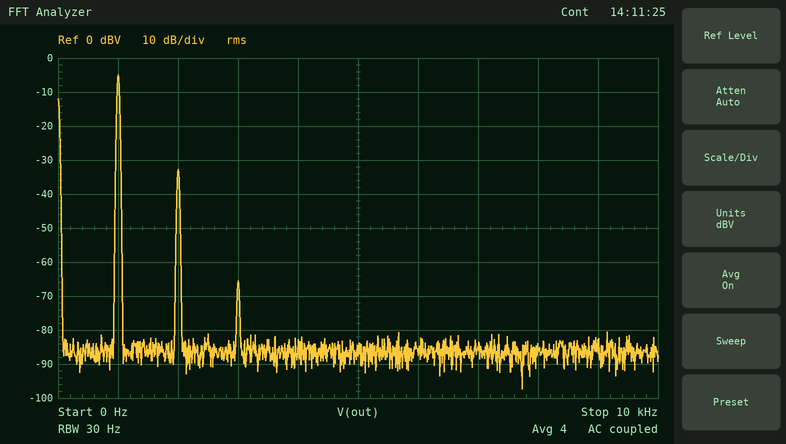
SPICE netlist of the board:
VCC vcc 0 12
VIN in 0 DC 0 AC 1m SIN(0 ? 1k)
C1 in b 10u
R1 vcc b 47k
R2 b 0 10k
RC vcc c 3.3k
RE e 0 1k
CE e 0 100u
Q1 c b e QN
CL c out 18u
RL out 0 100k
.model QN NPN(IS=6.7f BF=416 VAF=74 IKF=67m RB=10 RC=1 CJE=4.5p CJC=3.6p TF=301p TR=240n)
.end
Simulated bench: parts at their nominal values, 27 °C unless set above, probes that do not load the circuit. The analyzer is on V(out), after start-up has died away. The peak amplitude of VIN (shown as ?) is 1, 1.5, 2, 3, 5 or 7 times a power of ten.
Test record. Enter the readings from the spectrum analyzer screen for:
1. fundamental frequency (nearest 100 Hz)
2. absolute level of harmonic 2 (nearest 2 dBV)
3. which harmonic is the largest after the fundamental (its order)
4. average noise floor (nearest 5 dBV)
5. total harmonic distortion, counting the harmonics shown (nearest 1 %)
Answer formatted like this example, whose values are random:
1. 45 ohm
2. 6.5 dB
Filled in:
1. 1.0 kHz
2. -32 dBV
3. 2
4. -85 dBV
5. 4 %
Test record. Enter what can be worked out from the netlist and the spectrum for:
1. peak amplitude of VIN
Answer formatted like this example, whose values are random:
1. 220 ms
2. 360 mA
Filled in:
1. 5 mV
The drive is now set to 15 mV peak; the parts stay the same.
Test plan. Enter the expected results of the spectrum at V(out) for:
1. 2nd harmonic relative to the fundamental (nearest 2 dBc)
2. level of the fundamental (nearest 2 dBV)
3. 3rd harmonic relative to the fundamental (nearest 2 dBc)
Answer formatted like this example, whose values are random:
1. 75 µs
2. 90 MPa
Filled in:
1. -18 dBc
2. 4 dBV
3. -42 dBc
